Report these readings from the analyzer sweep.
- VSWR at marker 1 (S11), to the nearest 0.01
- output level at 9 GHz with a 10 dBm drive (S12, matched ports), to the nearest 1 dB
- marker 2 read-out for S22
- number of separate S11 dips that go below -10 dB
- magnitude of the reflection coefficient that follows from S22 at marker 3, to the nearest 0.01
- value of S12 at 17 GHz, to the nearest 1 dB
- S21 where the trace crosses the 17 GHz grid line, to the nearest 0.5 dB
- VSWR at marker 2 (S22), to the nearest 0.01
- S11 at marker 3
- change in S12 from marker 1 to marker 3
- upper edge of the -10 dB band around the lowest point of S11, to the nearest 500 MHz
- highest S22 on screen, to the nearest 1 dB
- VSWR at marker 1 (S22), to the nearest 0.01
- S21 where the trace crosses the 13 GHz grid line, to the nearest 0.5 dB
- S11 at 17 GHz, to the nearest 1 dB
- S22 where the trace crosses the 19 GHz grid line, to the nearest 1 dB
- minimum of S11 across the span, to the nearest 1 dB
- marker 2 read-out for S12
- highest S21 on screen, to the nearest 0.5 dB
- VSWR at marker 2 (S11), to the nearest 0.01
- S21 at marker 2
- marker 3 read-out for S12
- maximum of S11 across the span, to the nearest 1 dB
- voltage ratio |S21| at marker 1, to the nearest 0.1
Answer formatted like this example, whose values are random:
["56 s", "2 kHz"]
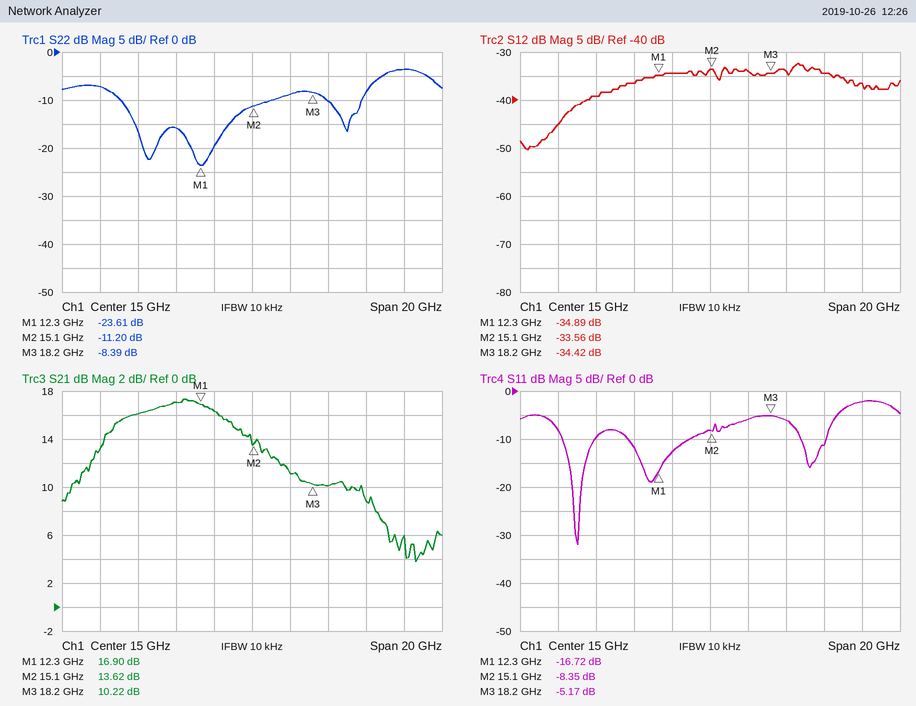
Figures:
["1.34", "-29 dBm", "-11.20 dB", "3", "0.38", "-34 dB", "11.0 dB", "1.76", "-5.17 dB", "0.47 dB", "9.0 GHz", "-4 dB", "1.14", "16.5 dB", "-6 dB", "-10 dB", "-32 dB", "-33.56 dB", "17.5 dB", "2.24", "13.62 dB", "-34.42 dB", "-2 dB", "7.0"]
